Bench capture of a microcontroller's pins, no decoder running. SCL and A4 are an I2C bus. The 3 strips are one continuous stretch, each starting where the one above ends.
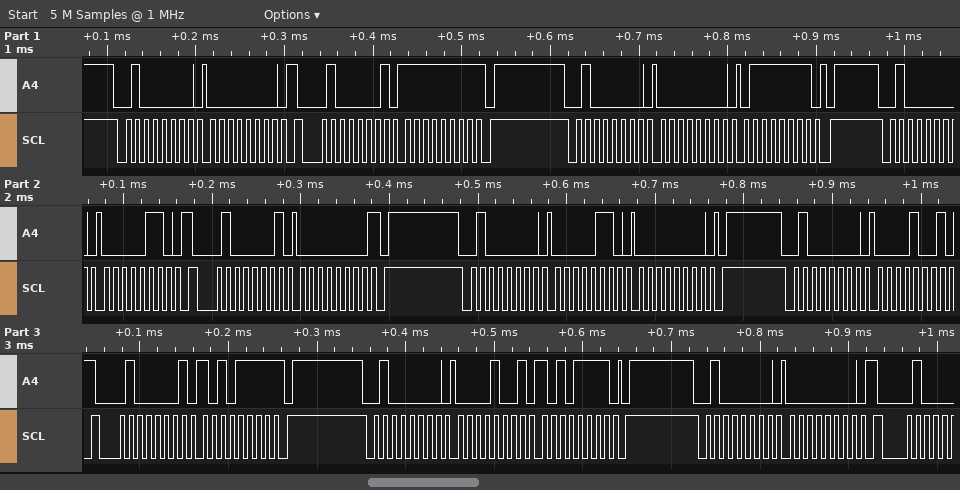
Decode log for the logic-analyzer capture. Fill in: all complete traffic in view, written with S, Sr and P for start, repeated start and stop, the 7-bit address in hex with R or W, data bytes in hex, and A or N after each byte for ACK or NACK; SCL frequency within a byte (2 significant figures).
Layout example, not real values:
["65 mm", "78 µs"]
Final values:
["S 20W A 00 A Sr 20R A FF N P S 20W A 00 A 7F A P S 20W A 06 A Sr 20R A 00 N P S 20W A 06 A 00 A P S 20W A 09 A Sr 20R A AF N P S 20W A 09 A AF A P S 20W A 00 A", "100 kHz"]
